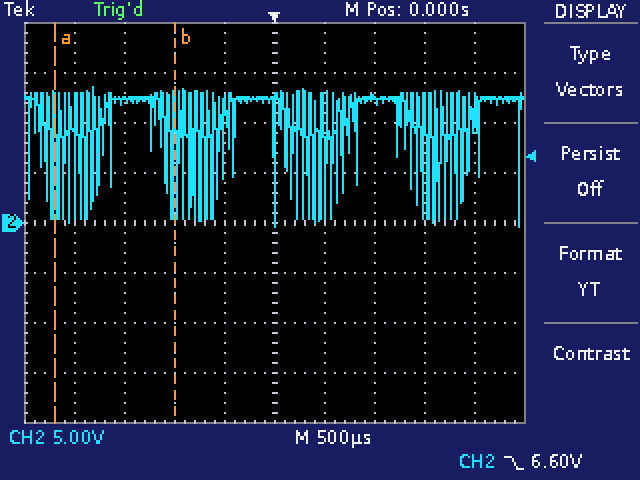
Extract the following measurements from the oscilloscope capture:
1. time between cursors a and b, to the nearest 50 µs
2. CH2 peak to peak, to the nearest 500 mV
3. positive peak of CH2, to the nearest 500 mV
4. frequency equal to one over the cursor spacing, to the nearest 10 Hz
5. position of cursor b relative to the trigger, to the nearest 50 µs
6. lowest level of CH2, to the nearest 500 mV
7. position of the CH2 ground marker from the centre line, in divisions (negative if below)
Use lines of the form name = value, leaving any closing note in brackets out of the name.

time between cursors a and b, to the nearest 50 µs = 1.20 ms
CH2 peak to peak, to the nearest 500 mV = 14.0 V
positive peak of CH2, to the nearest 500 mV = 13.5 V
frequency equal to one over the cursor spacing, to the nearest 10 Hz = 830 Hz
position of cursor b relative to the trigger, to the nearest 50 µs = -1.00 ms
lowest level of CH2, to the nearest 500 mV = -500 mV
position of the CH2 ground marker from the centre line, in divisions = 0.0 div
